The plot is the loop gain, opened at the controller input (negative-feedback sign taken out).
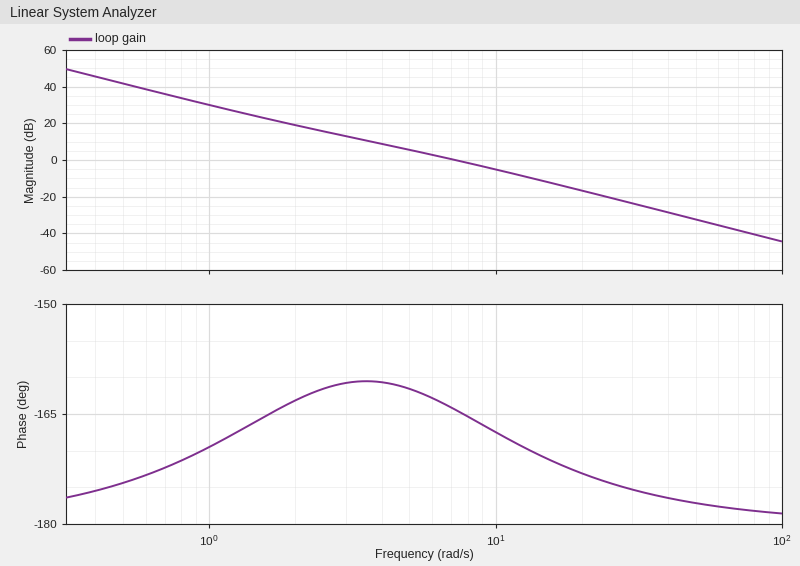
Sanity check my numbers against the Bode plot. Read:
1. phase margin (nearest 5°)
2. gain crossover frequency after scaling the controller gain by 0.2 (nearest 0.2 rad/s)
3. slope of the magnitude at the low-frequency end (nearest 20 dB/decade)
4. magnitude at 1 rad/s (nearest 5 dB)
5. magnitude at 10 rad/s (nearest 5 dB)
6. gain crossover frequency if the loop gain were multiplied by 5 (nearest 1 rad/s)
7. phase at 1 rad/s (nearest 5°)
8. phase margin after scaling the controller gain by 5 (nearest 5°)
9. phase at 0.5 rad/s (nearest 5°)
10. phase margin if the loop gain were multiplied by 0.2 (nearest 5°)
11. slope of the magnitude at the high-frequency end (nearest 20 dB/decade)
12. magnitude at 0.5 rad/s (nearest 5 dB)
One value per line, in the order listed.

15°
2.8 rad/s
-40 dB/decade
30 dB
-5 dB
17 rad/s
-170°
10°
-175°
20°
-40 dB/decade
40 dB
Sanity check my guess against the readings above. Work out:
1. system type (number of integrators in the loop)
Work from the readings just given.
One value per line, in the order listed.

2
